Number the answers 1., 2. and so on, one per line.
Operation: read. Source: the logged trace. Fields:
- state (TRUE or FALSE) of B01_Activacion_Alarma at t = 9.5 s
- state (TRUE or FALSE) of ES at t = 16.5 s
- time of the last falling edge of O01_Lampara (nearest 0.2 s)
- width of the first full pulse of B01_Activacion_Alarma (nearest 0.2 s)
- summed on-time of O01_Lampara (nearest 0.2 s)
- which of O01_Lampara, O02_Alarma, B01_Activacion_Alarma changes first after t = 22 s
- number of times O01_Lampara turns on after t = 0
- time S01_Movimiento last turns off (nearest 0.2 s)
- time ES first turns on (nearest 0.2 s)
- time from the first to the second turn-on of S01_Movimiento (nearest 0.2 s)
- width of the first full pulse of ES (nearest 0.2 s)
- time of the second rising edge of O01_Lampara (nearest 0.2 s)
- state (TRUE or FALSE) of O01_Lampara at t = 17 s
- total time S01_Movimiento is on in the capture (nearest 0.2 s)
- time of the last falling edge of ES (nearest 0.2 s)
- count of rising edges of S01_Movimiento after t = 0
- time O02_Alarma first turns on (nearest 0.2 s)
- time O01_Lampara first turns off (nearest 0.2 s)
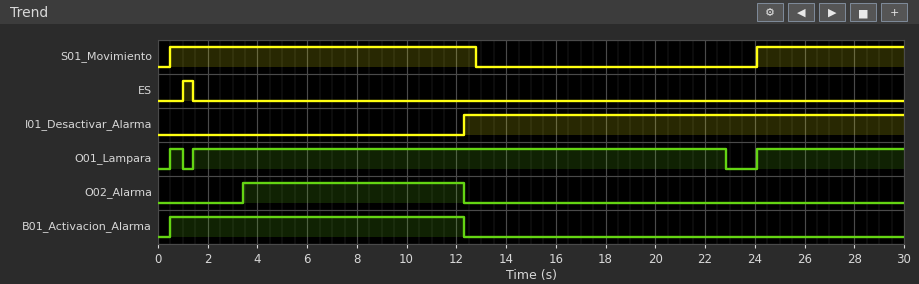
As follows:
1. TRUE
2. FALSE
3. 22.8 s
4. 11.8 s
5. 27.8 s
6. O01_Lampara
7. 3
8. 12.8 s
9. 1.0 s
10. 23.6 s
11. 0.4 s
12. 1.4 s
13. TRUE
14. 18.2 s
15. 1.4 s
16. 2
17. 3.4 s
18. 1.0 s
